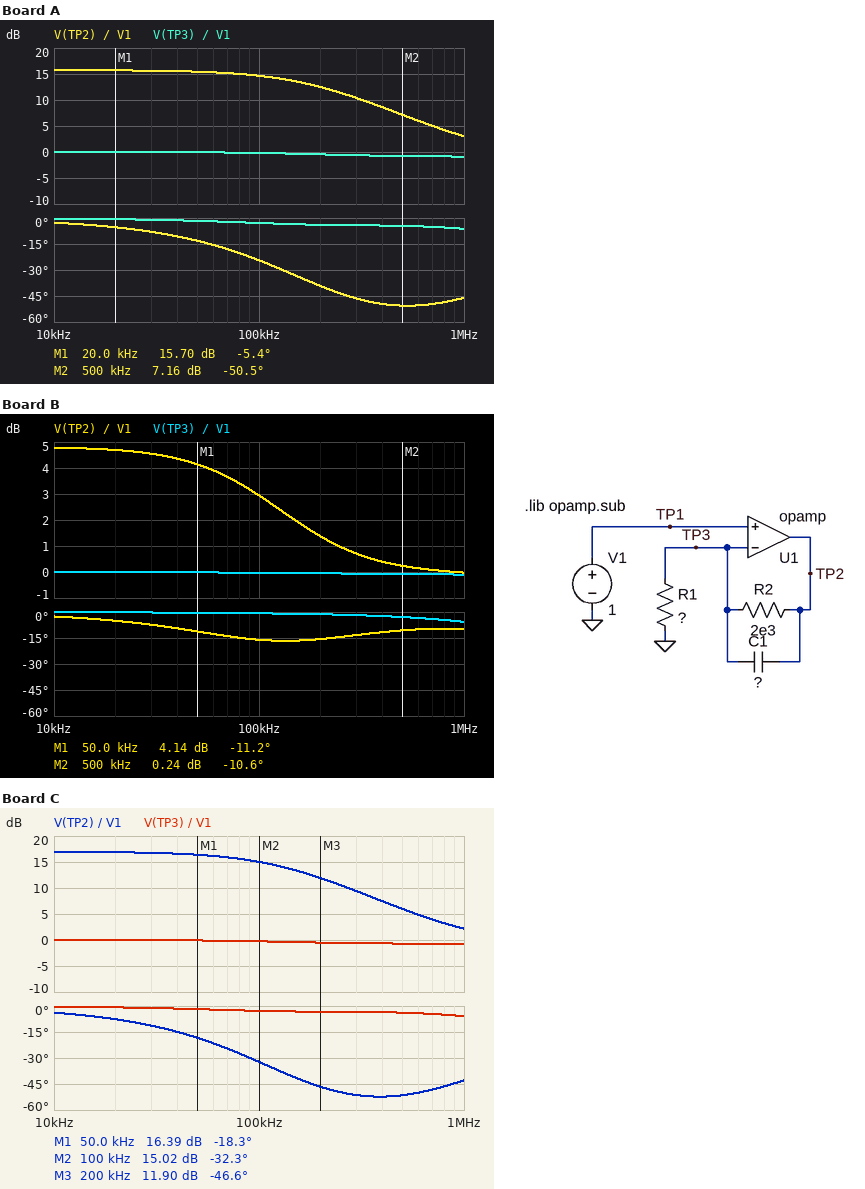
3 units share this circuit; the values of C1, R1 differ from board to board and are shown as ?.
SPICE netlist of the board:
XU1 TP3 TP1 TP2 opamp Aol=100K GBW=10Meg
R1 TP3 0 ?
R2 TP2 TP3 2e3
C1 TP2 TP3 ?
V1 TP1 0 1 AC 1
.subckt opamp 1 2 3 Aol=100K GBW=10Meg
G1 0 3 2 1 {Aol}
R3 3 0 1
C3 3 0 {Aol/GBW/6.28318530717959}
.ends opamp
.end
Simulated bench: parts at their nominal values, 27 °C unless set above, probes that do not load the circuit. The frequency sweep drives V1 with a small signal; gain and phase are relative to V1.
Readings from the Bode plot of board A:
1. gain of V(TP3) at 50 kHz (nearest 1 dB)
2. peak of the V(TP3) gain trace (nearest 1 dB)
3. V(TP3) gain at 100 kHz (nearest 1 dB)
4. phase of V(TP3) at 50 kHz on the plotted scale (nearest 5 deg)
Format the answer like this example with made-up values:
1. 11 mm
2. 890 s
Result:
1. 0 dB
2. 0 dB
3. 0 dB
4. 0 deg
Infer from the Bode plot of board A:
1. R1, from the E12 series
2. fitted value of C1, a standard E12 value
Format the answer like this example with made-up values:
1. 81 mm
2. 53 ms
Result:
1. 390 Ω
2. 390 pF
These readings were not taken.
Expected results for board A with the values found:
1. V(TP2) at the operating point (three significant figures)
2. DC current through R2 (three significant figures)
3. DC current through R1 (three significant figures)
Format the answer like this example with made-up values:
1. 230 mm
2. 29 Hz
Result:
1. 6.13 V
2. 2.56 mA
3. 2.56 mA
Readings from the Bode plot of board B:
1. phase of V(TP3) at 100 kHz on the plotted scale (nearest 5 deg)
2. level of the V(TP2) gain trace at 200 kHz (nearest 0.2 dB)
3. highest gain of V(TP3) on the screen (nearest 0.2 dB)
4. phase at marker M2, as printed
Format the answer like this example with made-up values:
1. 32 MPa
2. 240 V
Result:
1. 0 deg
2. 1.4 dB
3. 0 dB
4. -10.6 deg
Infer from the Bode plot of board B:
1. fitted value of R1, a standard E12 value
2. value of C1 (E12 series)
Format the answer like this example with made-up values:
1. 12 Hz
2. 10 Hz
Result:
1. 2.7 kΩ
2. 820 pF
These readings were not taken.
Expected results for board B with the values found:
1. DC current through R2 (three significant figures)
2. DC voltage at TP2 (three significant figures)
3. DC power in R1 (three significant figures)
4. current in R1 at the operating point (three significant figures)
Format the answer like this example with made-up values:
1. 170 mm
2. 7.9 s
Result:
1. 370 µA
2. 1.74 V
3. 370 µW
4. 370 µA
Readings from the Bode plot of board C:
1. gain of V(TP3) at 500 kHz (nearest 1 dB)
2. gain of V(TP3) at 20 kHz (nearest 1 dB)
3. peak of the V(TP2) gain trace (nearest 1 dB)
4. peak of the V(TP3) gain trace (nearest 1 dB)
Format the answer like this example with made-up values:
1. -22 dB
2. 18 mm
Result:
1. -1 dB
2. 0 dB
3. 17 dB
4. 0 dB
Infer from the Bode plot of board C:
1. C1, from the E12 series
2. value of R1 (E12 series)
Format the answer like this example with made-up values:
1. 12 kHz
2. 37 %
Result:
1. 560 pF
2. 330 Ω
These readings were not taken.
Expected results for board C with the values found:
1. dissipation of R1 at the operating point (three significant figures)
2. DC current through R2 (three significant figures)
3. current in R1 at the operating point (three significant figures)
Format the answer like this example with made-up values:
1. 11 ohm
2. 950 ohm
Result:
1. 3.03 mW
2. 3.03 mA
3. 3.03 mA
